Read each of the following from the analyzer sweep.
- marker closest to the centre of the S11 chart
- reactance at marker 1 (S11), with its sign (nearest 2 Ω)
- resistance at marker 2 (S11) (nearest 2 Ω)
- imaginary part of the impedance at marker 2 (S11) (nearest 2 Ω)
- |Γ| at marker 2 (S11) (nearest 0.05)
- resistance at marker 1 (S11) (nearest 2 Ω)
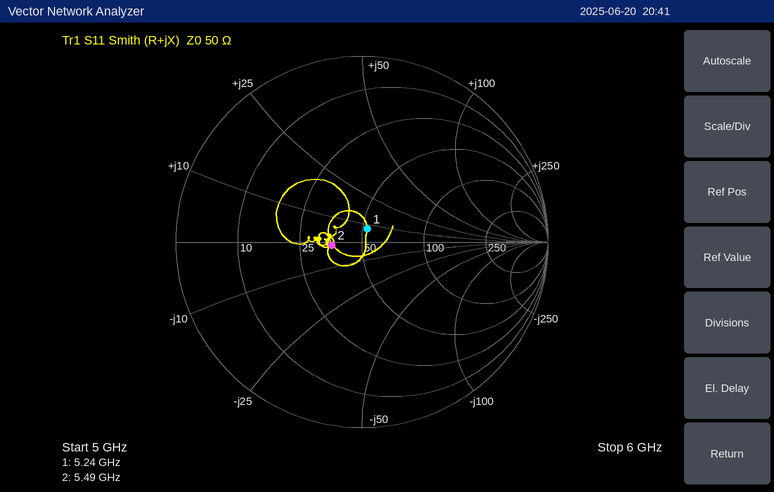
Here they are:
marker 1
+8 Ω
36 Ω
-2 Ω
0.15
52 Ω
